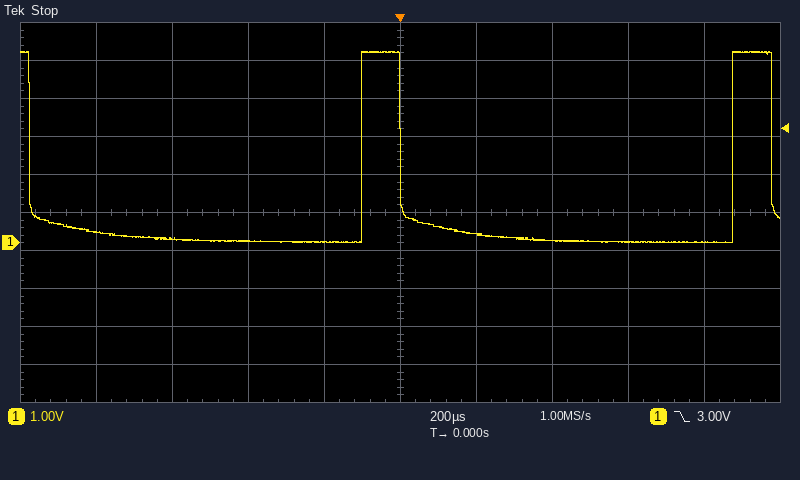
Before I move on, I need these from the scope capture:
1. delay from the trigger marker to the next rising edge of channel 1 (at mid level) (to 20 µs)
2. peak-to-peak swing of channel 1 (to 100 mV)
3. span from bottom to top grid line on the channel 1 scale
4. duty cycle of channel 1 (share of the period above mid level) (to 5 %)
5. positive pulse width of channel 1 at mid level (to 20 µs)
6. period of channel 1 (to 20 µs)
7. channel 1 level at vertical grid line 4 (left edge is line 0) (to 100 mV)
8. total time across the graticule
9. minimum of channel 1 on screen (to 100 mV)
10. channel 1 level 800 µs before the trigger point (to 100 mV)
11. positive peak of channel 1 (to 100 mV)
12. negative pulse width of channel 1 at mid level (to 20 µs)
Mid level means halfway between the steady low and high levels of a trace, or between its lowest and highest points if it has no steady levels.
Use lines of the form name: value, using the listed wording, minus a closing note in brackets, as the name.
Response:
delay from the trigger marker to the next rising edge of channel 1 (at mid level): 880 µs
peak-to-peak swing of channel 1: 5.0 V
span from bottom to top grid line on the channel 1 scale: 10 V
duty cycle of channel 1 (share of the period above mid level): 10 %
positive pulse width of channel 1 at mid level: 100 µs
period of channel 1: 980 µs
channel 1 level at vertical grid line 4 (left edge is line 0): 0.0 V
total time across the graticule: 2 ms
minimum of channel 1 on screen: 0.0 V
channel 1 level 800 µs before the trigger point: 300 mV
positive peak of channel 1: 5.0 V
negative pulse width of channel 1 at mid level: 880 µs
